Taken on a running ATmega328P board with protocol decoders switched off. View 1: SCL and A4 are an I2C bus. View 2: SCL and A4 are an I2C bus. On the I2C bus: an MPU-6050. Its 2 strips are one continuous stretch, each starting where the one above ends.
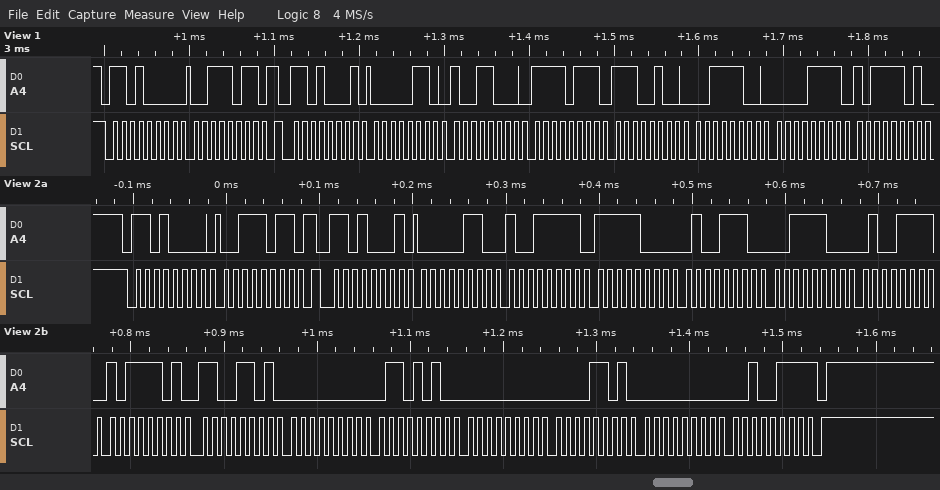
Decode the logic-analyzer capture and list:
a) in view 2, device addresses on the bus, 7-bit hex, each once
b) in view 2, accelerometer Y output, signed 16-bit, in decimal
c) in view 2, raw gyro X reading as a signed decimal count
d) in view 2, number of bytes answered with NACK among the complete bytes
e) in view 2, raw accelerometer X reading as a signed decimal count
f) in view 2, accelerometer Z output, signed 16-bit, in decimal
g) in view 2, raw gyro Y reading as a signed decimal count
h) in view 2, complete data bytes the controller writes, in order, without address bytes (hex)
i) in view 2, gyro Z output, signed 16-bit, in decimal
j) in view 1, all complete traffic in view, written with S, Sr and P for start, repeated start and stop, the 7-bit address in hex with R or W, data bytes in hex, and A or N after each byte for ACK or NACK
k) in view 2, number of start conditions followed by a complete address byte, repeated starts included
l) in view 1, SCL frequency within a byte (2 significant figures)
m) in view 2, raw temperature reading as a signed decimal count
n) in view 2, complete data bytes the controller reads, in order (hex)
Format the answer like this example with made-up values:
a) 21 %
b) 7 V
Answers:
a) 0x68
b) -1970
c) 106
d) 1
e) 1695
f) 15439
g) 13
h) 3B
i) 39
j) S 68W A 3B A Sr 68R A 06 A 98 A F7 A E4 A 3C A 0F A BD A
k) 2
l) 100 kHz
m) -16947
n) 06 9F F8 4E 3C 4F BD CD 00 6A 00 0D 00 27
